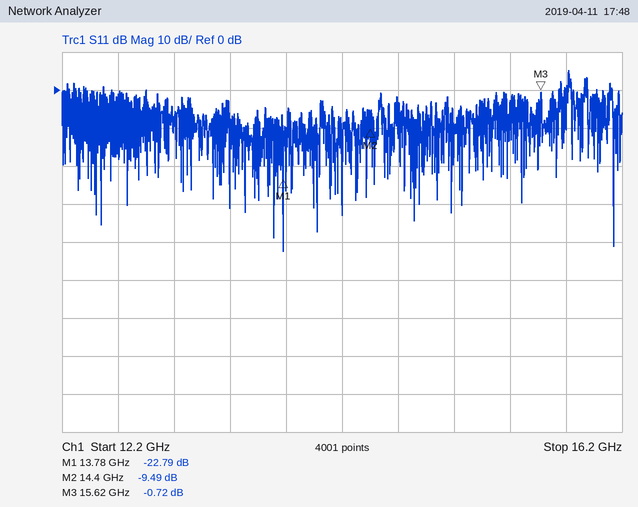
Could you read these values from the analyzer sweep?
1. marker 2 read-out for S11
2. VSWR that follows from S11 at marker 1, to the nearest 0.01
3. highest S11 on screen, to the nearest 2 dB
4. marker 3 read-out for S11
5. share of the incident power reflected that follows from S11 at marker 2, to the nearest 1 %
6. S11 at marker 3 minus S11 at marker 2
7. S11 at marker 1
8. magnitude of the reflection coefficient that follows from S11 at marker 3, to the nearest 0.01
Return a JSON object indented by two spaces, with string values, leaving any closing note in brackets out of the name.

{
  "marker 2 read-out for S11": "-9.49 dB",
  "VSWR that follows from S11 at marker 1, to the nearest 0.01": "1.16",
  "highest S11 on screen, to the nearest 2 dB": "6 dB",
  "marker 3 read-out for S11": "-0.72 dB",
  "share of the incident power reflected that follows from S11 at marker 2, to the nearest 1 %": "11 %",
  "S11 at marker 3 minus S11 at marker 2": "8.77 dB",
  "S11 at marker 1": "-22.79 dB",
  "magnitude of the reflection coefficient that follows from S11 at marker 3, to the nearest 0.01": "0.92"
}
